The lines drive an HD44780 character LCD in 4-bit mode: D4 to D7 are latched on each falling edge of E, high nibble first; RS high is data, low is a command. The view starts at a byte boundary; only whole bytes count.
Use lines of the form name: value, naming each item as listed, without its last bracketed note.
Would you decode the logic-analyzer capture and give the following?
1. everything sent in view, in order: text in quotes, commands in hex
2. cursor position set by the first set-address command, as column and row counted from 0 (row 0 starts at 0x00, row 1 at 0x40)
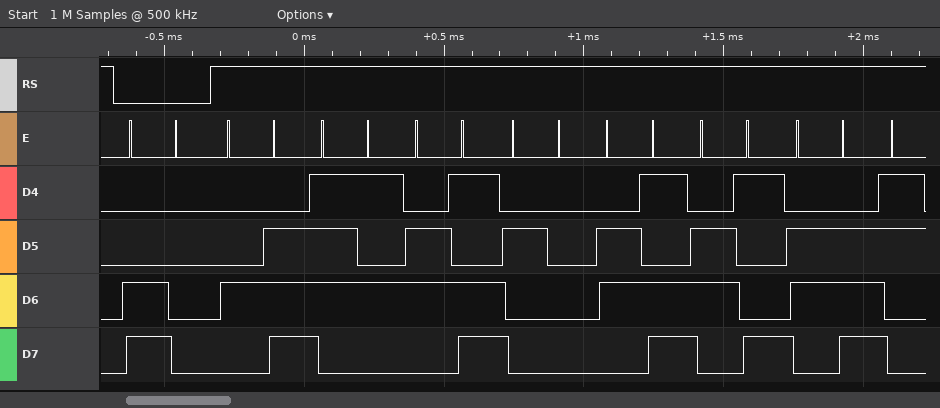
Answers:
everything sent in view, in order: text in quotes, commands in hex: 0xC0 "Num min"
cursor position set by the first set-address command, as column and row counted from 0: column 0, row 1
